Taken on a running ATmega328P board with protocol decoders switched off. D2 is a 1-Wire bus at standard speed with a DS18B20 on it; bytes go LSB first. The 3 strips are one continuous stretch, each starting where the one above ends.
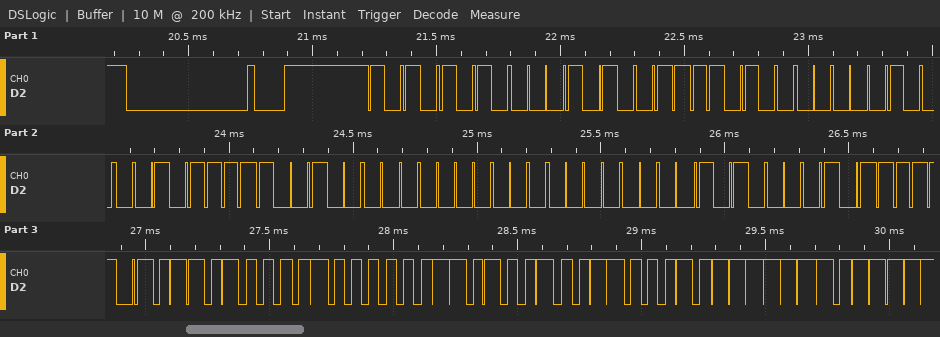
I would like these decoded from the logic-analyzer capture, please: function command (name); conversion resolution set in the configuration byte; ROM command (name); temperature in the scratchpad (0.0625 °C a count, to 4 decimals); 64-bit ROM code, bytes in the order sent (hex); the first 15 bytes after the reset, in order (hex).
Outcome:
Read Scratchpad
12 bits
Match ROM
33.3750 °C
28 2F 20 F4 09 00 00 85
55 28 2F 20 F4 09 00 00 85 BE 16 02 4B 46 7F
